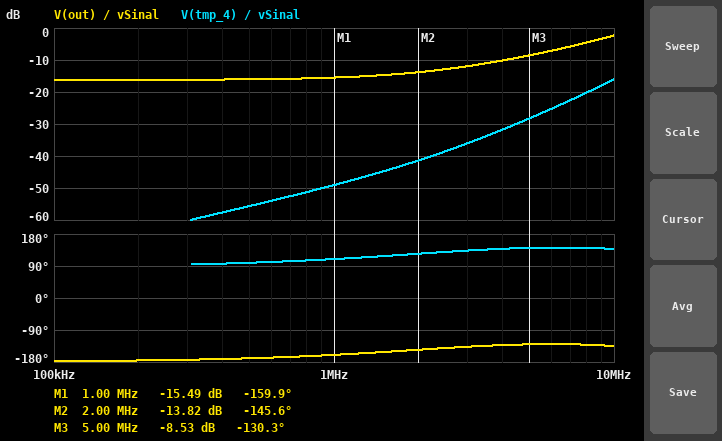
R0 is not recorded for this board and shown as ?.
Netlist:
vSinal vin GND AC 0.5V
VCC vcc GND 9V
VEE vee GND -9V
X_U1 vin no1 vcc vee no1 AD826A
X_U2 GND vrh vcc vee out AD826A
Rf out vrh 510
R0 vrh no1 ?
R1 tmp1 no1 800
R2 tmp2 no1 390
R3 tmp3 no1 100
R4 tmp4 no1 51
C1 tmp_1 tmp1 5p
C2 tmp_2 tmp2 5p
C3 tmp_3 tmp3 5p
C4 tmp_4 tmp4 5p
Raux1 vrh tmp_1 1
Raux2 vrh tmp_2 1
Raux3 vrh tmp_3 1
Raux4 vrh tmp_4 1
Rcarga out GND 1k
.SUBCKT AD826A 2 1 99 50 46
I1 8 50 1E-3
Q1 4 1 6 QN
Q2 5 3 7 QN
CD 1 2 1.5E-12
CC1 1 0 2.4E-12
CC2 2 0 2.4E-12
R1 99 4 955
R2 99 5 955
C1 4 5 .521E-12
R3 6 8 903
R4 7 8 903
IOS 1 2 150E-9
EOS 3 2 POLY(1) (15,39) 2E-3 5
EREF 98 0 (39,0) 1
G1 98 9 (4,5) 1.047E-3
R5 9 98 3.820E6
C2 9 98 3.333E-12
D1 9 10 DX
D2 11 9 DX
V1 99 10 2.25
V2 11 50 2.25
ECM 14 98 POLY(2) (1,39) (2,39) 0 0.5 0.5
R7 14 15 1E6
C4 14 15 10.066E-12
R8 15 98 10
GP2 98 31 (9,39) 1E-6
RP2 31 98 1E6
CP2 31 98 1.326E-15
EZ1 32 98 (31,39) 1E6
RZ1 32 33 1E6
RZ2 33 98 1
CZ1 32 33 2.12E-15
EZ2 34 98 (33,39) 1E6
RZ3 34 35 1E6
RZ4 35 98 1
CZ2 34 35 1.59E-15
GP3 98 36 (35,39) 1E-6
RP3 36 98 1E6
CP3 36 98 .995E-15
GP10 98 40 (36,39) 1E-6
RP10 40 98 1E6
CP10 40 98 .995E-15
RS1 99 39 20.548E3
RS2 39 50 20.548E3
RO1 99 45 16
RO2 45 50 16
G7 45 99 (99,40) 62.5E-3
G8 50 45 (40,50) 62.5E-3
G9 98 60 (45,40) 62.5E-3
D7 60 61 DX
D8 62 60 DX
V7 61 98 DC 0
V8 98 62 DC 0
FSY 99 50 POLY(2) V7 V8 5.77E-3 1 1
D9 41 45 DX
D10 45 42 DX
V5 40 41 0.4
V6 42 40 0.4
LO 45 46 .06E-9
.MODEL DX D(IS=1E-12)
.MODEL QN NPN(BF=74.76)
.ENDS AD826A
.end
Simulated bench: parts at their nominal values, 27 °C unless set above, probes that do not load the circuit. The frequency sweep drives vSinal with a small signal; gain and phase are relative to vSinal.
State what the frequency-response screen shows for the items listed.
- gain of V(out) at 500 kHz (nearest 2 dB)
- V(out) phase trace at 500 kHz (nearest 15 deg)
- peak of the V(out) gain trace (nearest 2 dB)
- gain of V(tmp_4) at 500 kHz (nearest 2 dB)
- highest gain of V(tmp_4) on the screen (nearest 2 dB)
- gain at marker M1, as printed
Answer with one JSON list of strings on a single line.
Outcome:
["-16 dB", "-165 deg", "-2 dB", "-56 dB", "-16 dB", "-15.49 dB"]
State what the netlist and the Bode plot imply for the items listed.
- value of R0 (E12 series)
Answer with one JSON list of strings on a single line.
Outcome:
["3.3 kΩ"]
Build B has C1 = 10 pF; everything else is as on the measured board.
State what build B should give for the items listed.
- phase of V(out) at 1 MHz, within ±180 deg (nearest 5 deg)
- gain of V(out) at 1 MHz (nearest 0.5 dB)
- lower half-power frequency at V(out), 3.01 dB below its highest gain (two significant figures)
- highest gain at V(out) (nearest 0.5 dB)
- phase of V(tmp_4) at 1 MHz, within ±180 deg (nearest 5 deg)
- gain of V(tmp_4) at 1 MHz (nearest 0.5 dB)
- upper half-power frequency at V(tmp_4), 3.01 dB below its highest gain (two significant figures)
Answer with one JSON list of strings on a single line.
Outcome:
["-155 deg", "-15.0 dB", "15 MHz", "7.0 dB", "115 deg", "-48.5 dB", "61 MHz"]
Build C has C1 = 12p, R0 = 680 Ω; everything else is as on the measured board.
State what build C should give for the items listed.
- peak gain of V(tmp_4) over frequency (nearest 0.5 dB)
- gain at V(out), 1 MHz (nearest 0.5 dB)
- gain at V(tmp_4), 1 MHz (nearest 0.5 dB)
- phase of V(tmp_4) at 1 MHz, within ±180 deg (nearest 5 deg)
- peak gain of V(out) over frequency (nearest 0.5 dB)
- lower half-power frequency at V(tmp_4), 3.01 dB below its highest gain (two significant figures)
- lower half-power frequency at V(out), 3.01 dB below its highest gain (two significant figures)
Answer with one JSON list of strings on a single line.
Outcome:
["-0.5 dB", "-2.5 dB", "-36.0 dB", "95 deg", "5.5 dB", "17 MHz", "10 MHz"]
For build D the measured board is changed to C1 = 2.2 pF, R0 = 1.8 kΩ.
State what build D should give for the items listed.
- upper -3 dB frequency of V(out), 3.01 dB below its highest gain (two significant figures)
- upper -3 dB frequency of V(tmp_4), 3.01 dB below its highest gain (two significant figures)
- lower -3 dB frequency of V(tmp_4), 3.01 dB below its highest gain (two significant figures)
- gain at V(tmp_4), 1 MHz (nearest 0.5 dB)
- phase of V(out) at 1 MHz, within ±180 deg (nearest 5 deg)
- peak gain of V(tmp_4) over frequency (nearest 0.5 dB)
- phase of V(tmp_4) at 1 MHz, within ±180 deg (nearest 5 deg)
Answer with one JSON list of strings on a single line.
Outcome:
["36 MHz", "54 MHz", "22 MHz", "-44.5 dB", "-170 deg", "1.5 dB", "100 deg"]
